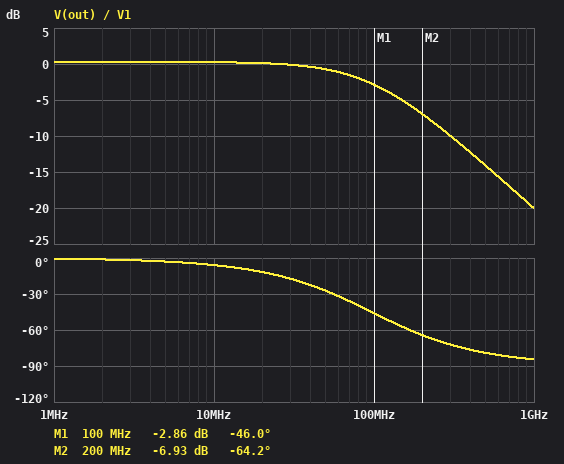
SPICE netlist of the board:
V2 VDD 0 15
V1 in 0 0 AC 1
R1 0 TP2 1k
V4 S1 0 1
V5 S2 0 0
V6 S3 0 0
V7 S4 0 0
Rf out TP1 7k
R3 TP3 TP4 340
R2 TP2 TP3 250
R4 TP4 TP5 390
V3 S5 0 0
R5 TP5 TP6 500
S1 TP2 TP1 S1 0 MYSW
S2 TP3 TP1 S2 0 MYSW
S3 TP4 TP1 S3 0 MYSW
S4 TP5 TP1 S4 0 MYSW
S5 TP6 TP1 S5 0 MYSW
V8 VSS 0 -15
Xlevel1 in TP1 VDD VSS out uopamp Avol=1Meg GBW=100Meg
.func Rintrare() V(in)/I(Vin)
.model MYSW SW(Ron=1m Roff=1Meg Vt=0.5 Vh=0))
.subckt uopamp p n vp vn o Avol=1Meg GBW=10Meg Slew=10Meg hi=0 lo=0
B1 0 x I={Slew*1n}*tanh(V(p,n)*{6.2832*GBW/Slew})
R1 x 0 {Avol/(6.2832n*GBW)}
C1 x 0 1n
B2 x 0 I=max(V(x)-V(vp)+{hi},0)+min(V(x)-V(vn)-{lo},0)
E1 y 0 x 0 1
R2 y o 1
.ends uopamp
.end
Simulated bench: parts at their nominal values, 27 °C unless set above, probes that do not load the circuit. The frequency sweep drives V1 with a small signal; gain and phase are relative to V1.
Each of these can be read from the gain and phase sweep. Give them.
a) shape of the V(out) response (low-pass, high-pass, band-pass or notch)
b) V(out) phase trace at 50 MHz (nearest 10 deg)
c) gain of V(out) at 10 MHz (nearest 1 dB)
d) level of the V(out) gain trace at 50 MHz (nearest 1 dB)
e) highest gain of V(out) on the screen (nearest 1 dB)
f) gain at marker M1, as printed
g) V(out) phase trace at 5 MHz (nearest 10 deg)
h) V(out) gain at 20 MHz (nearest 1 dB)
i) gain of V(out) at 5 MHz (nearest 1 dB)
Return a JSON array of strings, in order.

["low-pass", "-30 deg", "0 dB", "-1 dB", "0 dB", "-2.86 dB", "0 deg", "0 dB", "0 dB"]
